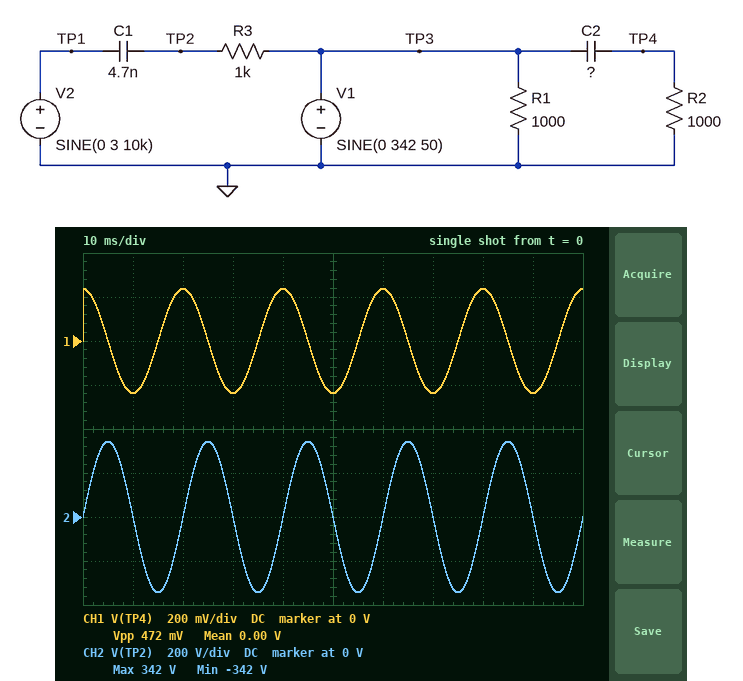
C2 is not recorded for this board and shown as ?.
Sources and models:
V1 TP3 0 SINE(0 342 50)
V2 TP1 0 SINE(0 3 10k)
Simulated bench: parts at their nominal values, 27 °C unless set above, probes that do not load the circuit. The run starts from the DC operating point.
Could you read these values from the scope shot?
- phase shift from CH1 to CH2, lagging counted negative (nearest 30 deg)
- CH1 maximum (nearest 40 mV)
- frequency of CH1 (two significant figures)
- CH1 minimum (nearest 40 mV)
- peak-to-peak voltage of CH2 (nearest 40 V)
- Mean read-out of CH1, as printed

-90 deg
240 mV
50 Hz
-240 mV
680 V
0.00 V
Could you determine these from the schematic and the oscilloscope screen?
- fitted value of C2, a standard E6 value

2.2 nF
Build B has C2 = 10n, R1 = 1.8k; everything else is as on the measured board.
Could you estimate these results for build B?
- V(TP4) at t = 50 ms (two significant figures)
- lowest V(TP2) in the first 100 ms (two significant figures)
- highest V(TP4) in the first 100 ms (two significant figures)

-1.1 V
-340 V
1.1 V
